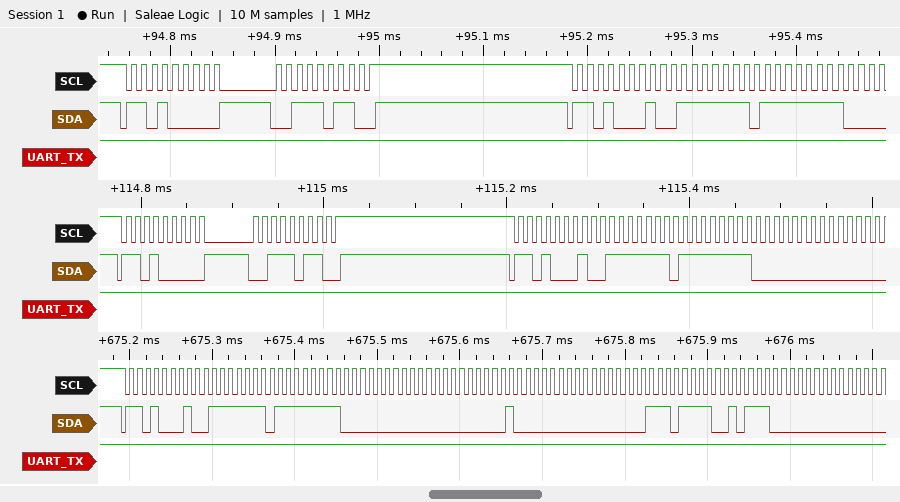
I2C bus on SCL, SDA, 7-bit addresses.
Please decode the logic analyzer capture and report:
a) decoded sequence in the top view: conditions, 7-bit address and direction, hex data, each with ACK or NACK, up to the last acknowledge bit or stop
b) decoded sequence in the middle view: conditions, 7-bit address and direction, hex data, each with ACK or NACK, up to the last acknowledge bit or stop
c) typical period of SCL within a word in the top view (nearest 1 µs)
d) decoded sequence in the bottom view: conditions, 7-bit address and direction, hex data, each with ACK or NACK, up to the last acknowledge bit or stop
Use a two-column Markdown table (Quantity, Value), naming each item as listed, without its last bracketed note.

| Quantity | Value |
|---|---|
| decoded sequence in the top view: conditions, 7-bit address and direction, hex data, each with ACK or NACK, up to the last acknowledge bit or stop | start, address 68 write ACK, 3B ACK, stop, start, address 68 read ACK, 7F ACK, FF ACK |
| decoded sequence in the middle view: conditions, 7-bit address and direction, hex data, each with ACK or NACK, up to the last acknowledge bit or stop | start, address 68 write ACK, 3B ACK, stop, start, address 68 read ACK, 7F ACK, FF ACK, 00 ACK |
| typical period of SCL within a word in the top view | 10 µs |
| decoded sequence in the bottom view: conditions, 7-bit address and direction, hex data, each with ACK or NACK, up to the last acknowledge bit or stop | start, address 68 read ACK, 7F ACK, FF ACK, 00 ACK, 00 ACK, 40 ACK, 00 ACK, EF ACK, 5C ACK, 00 ACK |
